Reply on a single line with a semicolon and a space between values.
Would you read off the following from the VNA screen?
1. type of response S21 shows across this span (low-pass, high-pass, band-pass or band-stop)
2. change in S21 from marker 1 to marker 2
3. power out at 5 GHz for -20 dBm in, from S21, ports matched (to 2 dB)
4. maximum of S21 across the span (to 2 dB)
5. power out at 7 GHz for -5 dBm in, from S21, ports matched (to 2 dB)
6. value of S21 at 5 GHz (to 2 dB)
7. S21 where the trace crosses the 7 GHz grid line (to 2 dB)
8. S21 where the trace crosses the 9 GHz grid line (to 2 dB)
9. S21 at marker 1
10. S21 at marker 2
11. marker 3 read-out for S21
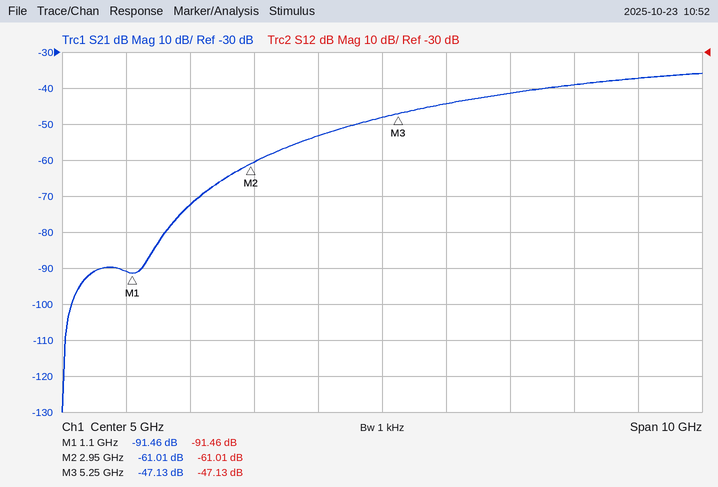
high-pass; 30.45 dB; -68 dBm; -36 dB; -46 dBm; -48 dB; -42 dB; -38 dB; -91.46 dB; -61.01 dB; -47.13 dB
